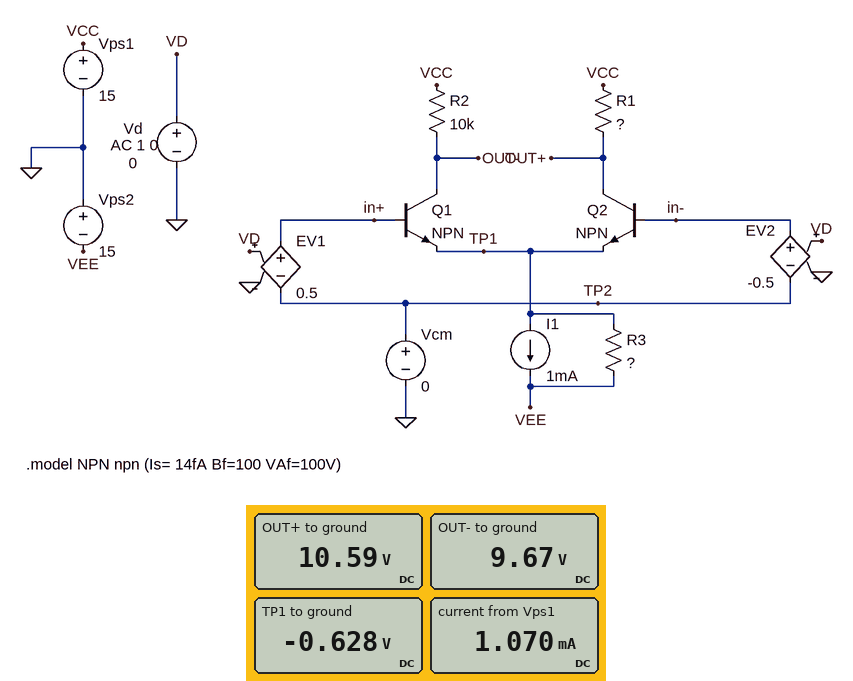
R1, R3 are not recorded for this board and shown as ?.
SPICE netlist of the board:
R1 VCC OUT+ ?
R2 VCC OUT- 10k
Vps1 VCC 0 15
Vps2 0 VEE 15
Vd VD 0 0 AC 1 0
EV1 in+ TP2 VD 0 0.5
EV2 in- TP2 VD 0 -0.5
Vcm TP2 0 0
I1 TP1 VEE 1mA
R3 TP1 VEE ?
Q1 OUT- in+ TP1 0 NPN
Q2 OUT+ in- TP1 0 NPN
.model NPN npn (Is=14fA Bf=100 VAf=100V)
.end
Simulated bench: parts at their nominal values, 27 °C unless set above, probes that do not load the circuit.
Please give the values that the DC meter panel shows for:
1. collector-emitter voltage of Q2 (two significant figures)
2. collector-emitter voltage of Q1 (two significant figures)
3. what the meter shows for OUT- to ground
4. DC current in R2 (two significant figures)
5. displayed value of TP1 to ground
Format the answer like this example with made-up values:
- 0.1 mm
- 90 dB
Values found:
- 11 V
- 10 V
- 9.67 V
- 530 µA
- -0.628 V
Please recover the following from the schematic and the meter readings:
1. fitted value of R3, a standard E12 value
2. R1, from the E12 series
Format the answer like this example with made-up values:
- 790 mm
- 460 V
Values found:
- 180 kΩ
- 8.2 kΩ
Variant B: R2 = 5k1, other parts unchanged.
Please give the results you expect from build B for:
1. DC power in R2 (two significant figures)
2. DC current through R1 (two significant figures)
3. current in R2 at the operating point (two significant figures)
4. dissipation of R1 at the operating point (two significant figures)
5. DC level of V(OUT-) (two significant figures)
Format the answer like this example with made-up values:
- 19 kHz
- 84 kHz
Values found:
- 1.5 mW
- 530 µA
- 540 µA
- 2.3 mW
- 12 V
